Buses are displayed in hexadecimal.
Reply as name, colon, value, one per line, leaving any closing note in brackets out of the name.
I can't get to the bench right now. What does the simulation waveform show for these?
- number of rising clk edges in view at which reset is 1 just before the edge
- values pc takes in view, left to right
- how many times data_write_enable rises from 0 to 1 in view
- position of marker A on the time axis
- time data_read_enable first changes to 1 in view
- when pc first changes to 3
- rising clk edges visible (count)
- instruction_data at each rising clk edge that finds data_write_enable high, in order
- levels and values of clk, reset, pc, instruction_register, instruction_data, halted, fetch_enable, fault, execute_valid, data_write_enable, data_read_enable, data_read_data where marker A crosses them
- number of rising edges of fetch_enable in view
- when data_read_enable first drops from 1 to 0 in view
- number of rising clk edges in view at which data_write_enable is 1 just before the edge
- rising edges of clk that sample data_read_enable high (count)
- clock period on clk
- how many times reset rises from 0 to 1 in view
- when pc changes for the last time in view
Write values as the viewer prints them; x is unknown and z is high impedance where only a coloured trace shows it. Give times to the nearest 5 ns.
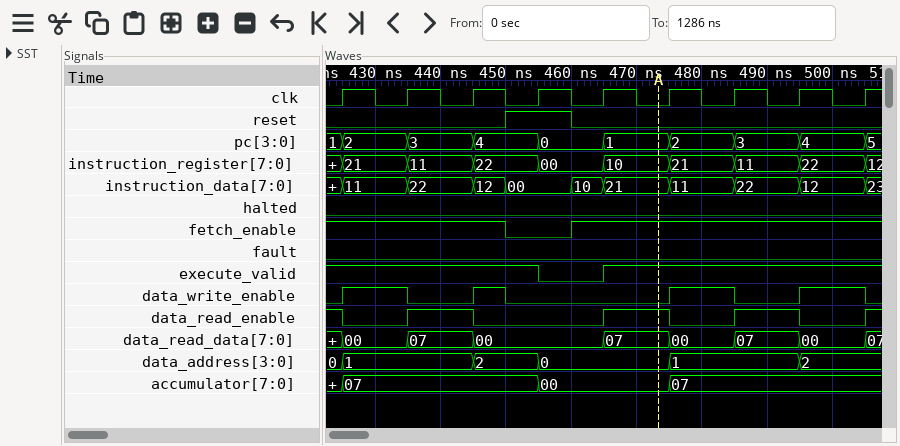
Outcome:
number of rising clk edges in view at which reset is 1 just before the edge: 1
values pc takes in view, left to right: 1, 2, 3, 4, 0, 1, 2, 3, 4, 5
how many times data_write_enable rises from 0 to 1 in view: 4
position of marker A on the time axis: 475 ns
time data_read_enable first changes to 1 in view: 435 ns
when pc first changes to 3: 435 ns
rising clk edges visible: 9
instruction_data at each rising clk edge that finds data_write_enable high, in order: 11, 11, 12
levels and values of clk, reset, pc, instruction_register, instruction_data, halted, fetch_enable, fault, execute_valid, data_write_enable, data_read_enable, data_read_data where marker A crosses them: clk=0, reset=0, pc=1, instruction_register=10, instruction_data=21, halted=0, fetch_enable=1, fault=0, execute_valid=1, data_write_enable=0, data_read_enable=1, data_read_data=07
number of rising edges of fetch_enable in view: 1
when data_read_enable first drops from 1 to 0 in view: 425 ns
number of rising clk edges in view at which data_write_enable is 1 just before the edge: 3
rising edges of clk that sample data_read_enable high: 4
clock period on clk: 10 ns
how many times reset rises from 0 to 1 in view: 1
when pc changes for the last time in view: 505 ns
